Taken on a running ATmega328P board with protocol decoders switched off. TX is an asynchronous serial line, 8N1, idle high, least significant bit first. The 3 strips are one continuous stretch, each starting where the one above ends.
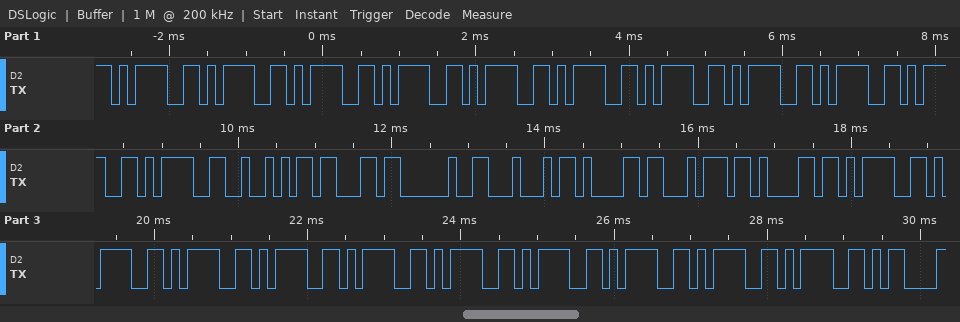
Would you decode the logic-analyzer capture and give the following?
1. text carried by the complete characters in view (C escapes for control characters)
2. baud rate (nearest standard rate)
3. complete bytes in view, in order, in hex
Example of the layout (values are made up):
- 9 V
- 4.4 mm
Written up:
- "===========Rc Data==========\r"
- 9600 baud
- 0x3D 0x3D 0x3D 0x3D 0x3D 0x3D 0x3D 0x3D 0x3D 0x3D 0x3D 0x52 0x63 0x20 0x44 0x61 0x74 0x61 0x3D 0x3D 0x3D 0x3D 0x3D 0x3D 0x3D 0x3D 0x3D 0x3D 0x0D
